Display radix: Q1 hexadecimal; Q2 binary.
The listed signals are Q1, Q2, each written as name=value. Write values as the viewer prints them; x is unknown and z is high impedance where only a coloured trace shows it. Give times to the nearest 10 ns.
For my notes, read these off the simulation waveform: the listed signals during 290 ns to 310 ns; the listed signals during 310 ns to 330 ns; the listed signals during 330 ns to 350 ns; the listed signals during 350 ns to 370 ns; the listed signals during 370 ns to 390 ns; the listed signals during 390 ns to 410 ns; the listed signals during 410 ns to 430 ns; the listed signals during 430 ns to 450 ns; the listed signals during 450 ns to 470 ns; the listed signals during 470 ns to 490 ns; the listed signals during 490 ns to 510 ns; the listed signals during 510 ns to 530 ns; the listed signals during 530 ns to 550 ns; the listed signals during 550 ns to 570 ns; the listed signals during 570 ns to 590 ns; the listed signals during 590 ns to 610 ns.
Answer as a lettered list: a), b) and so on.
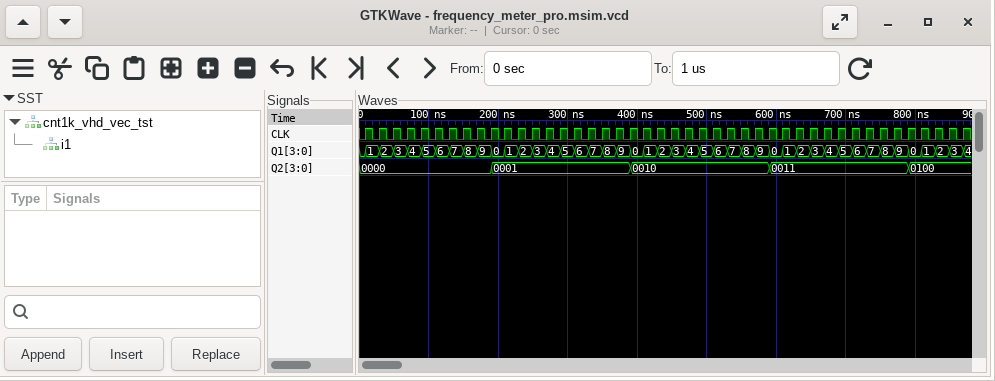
a) Q1=5, Q2=0001
b) Q1=6, Q2=0001
c) Q1=7, Q2=0001
d) Q1=8, Q2=0001
e) Q1=9, Q2=0001
f) Q1=0, Q2=0010
g) Q1=1, Q2=0010
h) Q1=2, Q2=0010
i) Q1=3, Q2=0010
j) Q1=4, Q2=0010
k) Q1=5, Q2=0010
l) Q1=6, Q2=0010
m) Q1=7, Q2=0010
n) Q1=8, Q2=0010
o) Q1=9, Q2=0010
p) Q1=0, Q2=0011
